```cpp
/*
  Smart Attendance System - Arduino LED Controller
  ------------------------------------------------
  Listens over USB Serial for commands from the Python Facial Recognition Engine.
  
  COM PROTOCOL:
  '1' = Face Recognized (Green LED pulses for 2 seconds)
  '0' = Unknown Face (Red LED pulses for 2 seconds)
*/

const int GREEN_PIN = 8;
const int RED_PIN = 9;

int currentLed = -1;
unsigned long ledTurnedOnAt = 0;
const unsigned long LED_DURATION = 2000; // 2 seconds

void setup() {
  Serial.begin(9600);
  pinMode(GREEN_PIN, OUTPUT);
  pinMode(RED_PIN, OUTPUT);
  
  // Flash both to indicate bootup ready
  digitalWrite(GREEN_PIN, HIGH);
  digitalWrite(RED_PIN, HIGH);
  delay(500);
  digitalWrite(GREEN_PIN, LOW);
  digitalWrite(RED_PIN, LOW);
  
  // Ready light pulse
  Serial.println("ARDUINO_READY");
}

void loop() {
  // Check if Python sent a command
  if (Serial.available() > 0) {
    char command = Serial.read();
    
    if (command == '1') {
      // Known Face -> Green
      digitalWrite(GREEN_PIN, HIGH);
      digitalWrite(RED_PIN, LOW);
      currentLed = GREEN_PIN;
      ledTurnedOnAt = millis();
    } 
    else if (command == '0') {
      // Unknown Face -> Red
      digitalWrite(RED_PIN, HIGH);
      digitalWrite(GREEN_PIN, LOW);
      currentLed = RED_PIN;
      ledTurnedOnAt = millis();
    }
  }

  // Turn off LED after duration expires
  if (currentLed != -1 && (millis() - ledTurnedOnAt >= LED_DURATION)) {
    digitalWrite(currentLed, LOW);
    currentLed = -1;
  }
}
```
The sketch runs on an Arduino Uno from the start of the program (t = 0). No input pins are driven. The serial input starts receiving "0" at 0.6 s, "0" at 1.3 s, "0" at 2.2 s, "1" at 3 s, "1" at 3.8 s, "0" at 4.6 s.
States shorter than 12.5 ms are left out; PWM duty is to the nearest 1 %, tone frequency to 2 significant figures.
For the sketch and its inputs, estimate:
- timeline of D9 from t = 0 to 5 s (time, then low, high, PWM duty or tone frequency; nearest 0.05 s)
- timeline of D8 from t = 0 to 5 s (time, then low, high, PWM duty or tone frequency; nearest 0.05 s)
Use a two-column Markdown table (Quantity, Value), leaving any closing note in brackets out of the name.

| Quantity | Value |
|---|---|
| timeline of D9 from t = 0 to 5 s | 0 s high; 0.5 s low; 0.6 s high; 3 s low; 4.6 s high |
| timeline of D8 from t = 0 to 5 s | 0 s high; 0.5 s low; 3 s high; 4.6 s low |
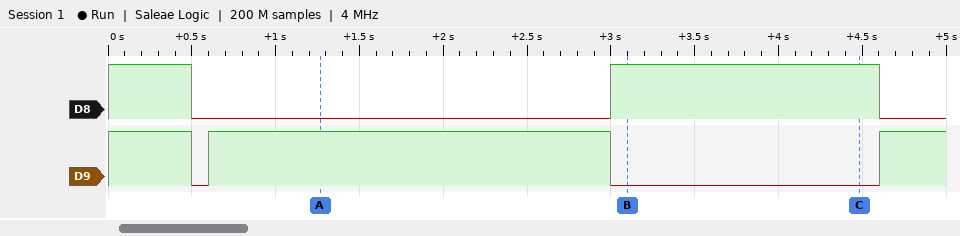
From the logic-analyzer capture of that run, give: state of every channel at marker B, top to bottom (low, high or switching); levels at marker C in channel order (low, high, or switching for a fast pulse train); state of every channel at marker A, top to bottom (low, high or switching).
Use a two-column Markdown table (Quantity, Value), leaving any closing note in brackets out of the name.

| Quantity | Value |
|---|---|
| state of every channel at marker B, top to bottom | D8 high, D9 low |
| levels at marker C in channel order | D8 high, D9 low |
| state of every channel at marker A, top to bottom | D8 low, D9 high |
